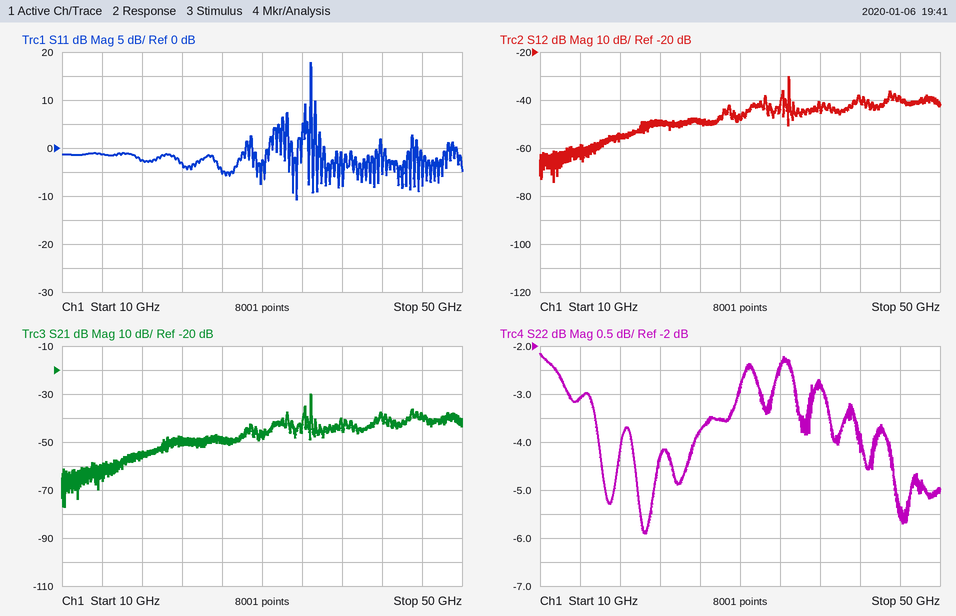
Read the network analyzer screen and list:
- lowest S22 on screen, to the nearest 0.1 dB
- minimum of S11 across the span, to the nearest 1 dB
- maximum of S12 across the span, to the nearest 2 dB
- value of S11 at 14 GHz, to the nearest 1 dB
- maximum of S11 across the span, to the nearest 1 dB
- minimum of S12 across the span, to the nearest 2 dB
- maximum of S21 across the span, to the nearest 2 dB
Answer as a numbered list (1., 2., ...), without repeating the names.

1. -5.9 dB
2. -11 dB
3. -30 dB
4. -1 dB
5. 18 dB
6. -74 dB
7. -30 dB
